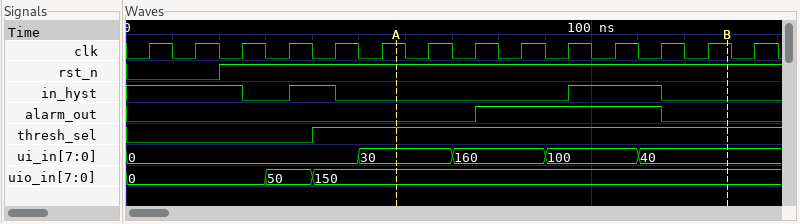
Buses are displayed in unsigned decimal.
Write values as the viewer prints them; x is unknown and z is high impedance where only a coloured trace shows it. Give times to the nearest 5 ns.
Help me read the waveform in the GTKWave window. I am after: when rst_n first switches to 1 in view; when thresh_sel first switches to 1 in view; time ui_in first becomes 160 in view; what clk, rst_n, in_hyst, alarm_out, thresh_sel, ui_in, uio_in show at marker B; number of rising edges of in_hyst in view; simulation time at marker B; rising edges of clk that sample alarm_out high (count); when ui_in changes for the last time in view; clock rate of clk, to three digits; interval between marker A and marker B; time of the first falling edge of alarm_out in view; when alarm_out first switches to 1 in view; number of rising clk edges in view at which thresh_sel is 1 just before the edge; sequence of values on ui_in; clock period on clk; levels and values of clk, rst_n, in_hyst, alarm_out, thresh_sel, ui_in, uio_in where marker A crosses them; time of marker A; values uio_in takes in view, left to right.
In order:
20 ns
40 ns
70 ns
clk=1, rst_n=1, in_hyst=0, alarm_out=0, thresh_sel=1, ui_in=40, uio_in=150
2
130 ns
4
110 ns
100 MHz
70 ns
115 ns
75 ns
10
0, 30, 160, 100, 40
10 ns
clk=1, rst_n=1, in_hyst=0, alarm_out=0, thresh_sel=1, ui_in=30, uio_in=150
60 ns
0, 50, 150
